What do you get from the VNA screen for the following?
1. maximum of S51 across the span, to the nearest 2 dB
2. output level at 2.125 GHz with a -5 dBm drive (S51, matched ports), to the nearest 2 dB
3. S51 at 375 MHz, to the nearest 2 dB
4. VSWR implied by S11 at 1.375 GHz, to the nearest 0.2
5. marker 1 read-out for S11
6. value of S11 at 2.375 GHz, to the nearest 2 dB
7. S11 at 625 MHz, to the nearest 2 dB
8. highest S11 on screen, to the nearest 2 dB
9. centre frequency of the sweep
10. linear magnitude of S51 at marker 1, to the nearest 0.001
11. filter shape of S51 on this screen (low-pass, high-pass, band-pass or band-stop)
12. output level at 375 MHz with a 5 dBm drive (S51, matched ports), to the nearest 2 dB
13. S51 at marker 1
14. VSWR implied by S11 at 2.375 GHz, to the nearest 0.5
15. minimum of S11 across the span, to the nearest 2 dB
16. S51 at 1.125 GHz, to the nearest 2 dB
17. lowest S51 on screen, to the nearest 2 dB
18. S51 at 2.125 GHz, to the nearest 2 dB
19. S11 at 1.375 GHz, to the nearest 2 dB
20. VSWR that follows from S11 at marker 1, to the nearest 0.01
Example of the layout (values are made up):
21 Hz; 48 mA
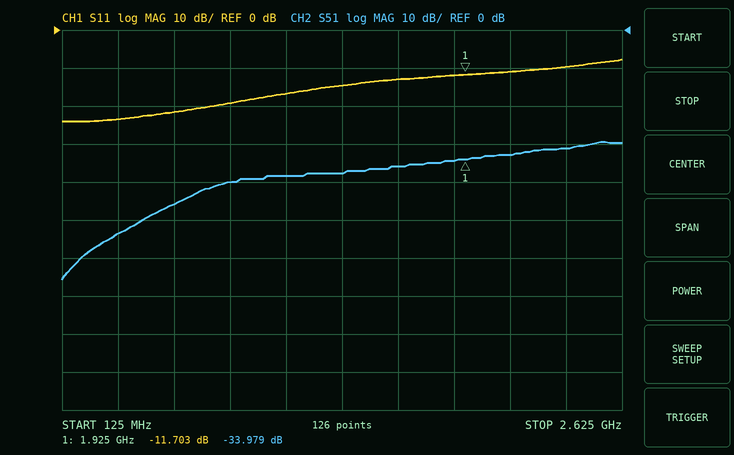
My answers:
-30 dB; -38 dBm; -54 dB; 1.4; -11.703 dB; -10 dB; -22 dB; -8 dB; 1.375 GHz; 0.020; high-pass; -48 dBm; -33.979 dB; 2.0; -24 dB; -38 dB; -66 dB; -32 dB; -14 dB; 1.70
